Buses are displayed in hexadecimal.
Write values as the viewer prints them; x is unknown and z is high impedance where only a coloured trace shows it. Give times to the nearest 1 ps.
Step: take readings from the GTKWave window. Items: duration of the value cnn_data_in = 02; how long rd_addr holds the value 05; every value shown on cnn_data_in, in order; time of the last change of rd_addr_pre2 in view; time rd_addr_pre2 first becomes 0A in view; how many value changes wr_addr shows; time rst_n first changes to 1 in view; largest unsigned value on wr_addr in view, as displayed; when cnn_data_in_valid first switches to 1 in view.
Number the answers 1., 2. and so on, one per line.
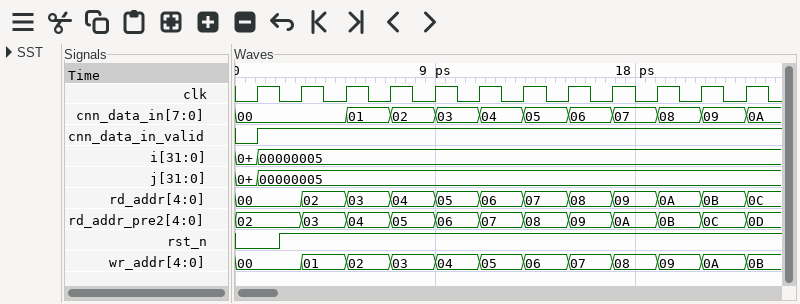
1. 2 ps
2. 2 ps
3. 00, 01, 02, 03, 04, 05, 06, 07, 08, 09, 0A
4. 23 ps
5. 17 ps
6. 11
7. 2 ps
8. 0B
9. 1 ps
